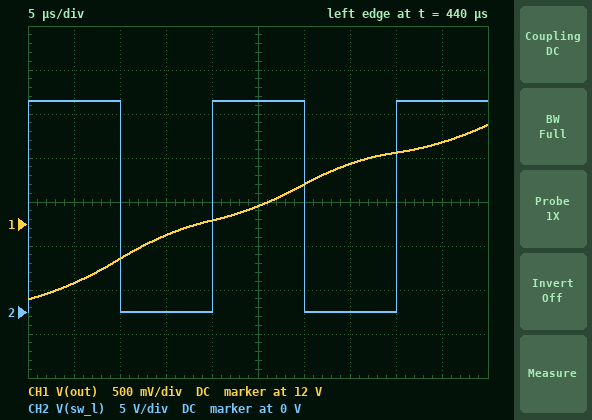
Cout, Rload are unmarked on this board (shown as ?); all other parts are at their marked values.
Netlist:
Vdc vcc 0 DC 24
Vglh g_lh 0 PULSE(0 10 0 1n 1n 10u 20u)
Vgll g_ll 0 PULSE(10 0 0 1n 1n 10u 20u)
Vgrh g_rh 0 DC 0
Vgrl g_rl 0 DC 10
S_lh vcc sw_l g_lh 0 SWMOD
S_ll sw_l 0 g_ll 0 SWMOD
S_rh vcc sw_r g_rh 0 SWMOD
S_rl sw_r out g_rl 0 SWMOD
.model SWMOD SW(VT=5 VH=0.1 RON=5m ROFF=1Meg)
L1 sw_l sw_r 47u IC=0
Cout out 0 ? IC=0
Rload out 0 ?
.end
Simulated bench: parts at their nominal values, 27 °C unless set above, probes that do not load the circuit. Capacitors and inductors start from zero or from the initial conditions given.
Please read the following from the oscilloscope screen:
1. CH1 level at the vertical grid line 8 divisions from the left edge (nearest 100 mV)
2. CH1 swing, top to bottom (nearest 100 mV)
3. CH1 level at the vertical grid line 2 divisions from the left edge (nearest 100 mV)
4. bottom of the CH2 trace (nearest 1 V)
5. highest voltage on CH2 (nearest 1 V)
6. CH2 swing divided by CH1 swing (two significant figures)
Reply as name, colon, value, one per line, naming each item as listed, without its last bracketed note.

CH1 level at the vertical grid line 8 divisions from the left edge: 12.8 V
CH1 swing, top to bottom: 2.0 V
CH1 level at the vertical grid line 2 divisions from the left edge: 11.6 V
bottom of the CH2 trace: 0 V
highest voltage on CH2: 24 V
CH2 swing divided by CH1 swing: 12
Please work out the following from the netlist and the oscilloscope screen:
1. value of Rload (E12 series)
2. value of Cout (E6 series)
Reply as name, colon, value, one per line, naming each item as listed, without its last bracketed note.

value of Rload: 2.2 Ω
value of Cout: 68 µF
